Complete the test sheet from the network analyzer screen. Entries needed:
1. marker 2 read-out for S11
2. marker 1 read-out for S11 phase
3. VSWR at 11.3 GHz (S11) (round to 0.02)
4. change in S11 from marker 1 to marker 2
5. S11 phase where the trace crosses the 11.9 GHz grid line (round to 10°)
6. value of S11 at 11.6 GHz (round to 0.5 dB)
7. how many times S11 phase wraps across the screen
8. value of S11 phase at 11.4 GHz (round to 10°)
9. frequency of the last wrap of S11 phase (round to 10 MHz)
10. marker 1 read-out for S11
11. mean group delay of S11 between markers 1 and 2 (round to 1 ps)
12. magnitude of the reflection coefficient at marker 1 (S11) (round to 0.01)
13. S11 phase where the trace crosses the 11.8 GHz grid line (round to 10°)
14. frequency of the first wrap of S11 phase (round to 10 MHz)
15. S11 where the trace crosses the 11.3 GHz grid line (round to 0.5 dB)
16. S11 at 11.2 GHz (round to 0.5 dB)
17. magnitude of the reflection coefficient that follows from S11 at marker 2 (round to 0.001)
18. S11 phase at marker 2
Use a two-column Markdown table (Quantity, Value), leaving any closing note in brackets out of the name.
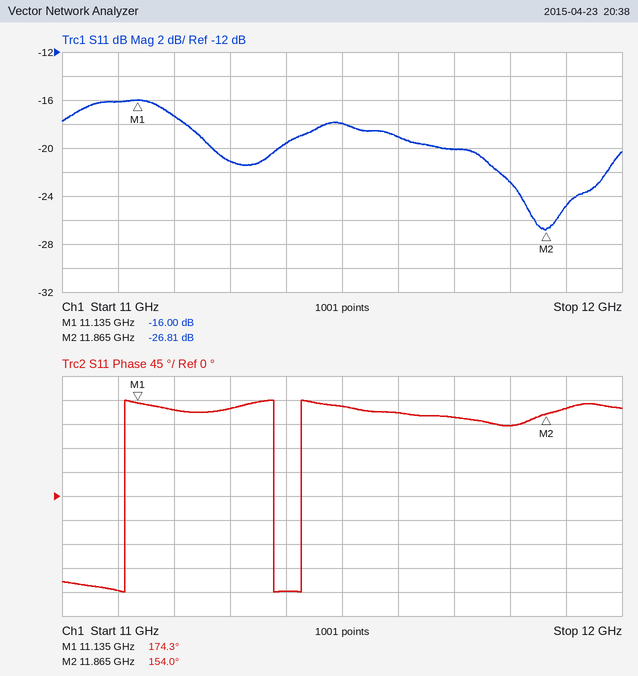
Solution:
| Quantity | Value |
|---|---|
| marker 2 read-out for S11 | -26.81 dB |
| marker 1 read-out for S11 phase | 174.3° |
| VSWR at 11.3 GHz (S11) | 1.20 |
| change in S11 from marker 1 to marker 2 | -10.81 dB |
| S11 phase where the trace crosses the 11.9 GHz grid line | 160° |
| value of S11 at 11.6 GHz | -19.0 dB |
| how many times S11 phase wraps across the screen | 3 |
| value of S11 phase at 11.4 GHz | -180° |
| frequency of the last wrap of S11 phase | 11.43 GHz |
| marker 1 read-out for S11 | -16.00 dB |
| mean group delay of S11 between markers 1 and 2 | 77 ps |
| magnitude of the reflection coefficient at marker 1 (S11) | 0.16 |
| S11 phase where the trace crosses the 11.8 GHz grid line | 130° |
| frequency of the first wrap of S11 phase | 11.11 GHz |
| S11 where the trace crosses the 11.3 GHz grid line | -21.0 dB |
| S11 at 11.2 GHz | -17.5 dB |
| magnitude of the reflection coefficient that follows from S11 at marker 2 | 0.046 |
| S11 phase at marker 2 | 154.0° |
